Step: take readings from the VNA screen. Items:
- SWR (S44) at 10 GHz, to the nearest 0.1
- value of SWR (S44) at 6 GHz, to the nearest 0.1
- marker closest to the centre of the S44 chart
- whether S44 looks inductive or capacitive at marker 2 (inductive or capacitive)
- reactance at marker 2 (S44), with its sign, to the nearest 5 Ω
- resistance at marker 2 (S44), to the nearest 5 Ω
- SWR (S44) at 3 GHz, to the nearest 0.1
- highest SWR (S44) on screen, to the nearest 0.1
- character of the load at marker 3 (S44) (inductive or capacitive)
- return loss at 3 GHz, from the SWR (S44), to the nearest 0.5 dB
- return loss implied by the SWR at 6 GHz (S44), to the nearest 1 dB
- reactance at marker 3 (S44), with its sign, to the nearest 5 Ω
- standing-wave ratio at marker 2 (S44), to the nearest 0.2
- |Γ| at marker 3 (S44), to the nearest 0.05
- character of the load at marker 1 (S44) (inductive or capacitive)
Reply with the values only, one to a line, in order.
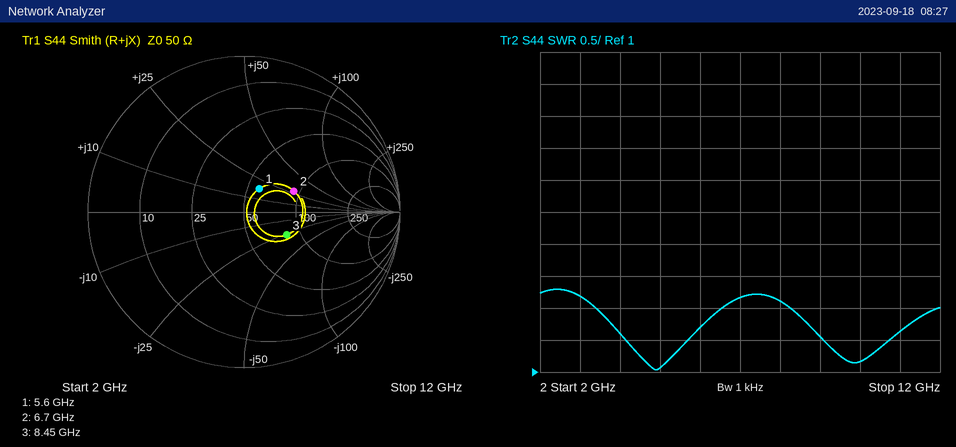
1.2
1.7
marker 1
inductive
+30 Ω
90 Ω
2.2
2.3
capacitive
8.5 dB
12 dB
-25 Ω
2.0
0.30
inductive
